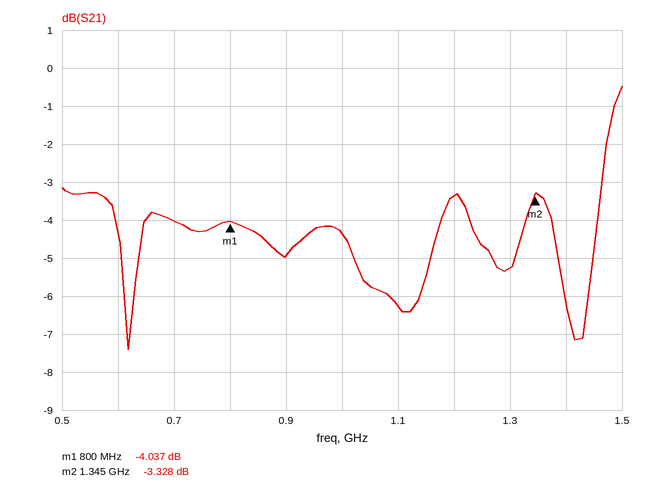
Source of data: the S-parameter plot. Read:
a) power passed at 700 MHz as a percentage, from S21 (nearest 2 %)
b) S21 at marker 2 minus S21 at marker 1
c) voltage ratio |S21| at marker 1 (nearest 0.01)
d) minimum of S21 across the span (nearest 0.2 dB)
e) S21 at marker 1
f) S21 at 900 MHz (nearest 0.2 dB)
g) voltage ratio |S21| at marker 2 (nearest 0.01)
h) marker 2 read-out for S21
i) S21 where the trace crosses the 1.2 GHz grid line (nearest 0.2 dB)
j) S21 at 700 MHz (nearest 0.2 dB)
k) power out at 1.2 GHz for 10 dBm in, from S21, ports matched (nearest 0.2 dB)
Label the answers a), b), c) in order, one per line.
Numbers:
a) 40 %
b) 0.709 dB
c) 0.63
d) -7.4 dB
e) -4.037 dB
f) -5.0 dB
g) 0.68
h) -3.328 dB
i) -3.4 dB
j) -4.0 dB
k) 6.6 dBm
